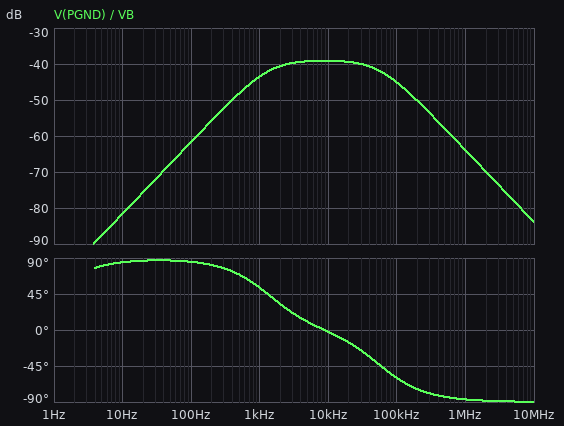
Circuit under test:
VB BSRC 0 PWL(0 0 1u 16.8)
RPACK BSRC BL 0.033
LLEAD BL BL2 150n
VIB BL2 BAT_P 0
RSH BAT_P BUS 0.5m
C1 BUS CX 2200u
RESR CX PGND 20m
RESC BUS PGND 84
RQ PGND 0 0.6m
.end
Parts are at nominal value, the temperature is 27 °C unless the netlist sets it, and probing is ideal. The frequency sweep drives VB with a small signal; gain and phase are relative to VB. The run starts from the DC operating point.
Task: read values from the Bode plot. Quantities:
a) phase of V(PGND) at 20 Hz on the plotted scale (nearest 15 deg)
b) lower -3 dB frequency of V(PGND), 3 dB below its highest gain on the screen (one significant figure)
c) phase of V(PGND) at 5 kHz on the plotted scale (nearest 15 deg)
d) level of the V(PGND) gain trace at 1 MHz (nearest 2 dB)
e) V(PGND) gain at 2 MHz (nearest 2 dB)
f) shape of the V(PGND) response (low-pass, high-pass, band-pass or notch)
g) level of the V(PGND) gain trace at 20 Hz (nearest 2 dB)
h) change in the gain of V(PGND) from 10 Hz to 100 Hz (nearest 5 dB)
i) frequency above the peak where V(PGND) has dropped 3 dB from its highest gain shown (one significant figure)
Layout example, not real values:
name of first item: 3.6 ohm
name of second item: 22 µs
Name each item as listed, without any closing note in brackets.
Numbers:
phase of V(PGND) at 20 Hz on the plotted scale: 90 deg
lower -3 dB frequency of V(PGND), 3 dB below its highest gain on the screen: 1 kHz
phase of V(PGND) at 5 kHz on the plotted scale: 15 deg
level of the V(PGND) gain trace at 1 MHz: -64 dB
V(PGND) gain at 2 MHz: -70 dB
shape of the V(PGND) response: band-pass
level of the V(PGND) gain trace at 20 Hz: -76 dB
change in the gain of V(PGND) from 10 Hz to 100 Hz: 20 dB
frequency above the peak where V(PGND) has dropped 3 dB from its highest gain shown: 60 kHz
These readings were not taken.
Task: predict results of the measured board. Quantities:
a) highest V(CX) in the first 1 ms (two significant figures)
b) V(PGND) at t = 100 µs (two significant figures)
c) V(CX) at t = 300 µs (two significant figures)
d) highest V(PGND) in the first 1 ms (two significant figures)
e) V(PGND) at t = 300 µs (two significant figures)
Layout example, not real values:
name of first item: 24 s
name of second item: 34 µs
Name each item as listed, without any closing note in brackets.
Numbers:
highest V(CX) in the first 1 ms: 6.0 V
V(PGND) at t = 100 µs: 83 mV
V(CX) at t = 300 µs: 510 mV
highest V(PGND) in the first 1 ms: 170 mV
V(PGND) at t = 300 µs: 15 mV
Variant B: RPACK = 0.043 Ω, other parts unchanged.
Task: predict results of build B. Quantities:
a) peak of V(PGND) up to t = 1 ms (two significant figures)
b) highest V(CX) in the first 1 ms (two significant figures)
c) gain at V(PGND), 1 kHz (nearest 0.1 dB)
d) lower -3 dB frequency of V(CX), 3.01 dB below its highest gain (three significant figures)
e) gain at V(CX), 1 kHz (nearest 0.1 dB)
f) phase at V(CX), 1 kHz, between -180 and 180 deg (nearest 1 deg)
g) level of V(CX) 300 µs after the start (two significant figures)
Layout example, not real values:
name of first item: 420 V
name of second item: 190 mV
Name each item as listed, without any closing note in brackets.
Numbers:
peak of V(PGND) up to t = 1 ms: 150 mV
highest V(CX) in the first 1 ms: 5.1 V
gain at V(PGND), 1 kHz: -44.1 dB
lower -3 dB frequency of V(CX), 3.01 dB below its highest gain: 1.11 kHz
gain at V(CX), 1 kHz: -13.4 dB
phase at V(CX), 1 kHz, between -180 and 180 deg: 48 deg
level of V(CX) 300 µs after the start: 640 mV
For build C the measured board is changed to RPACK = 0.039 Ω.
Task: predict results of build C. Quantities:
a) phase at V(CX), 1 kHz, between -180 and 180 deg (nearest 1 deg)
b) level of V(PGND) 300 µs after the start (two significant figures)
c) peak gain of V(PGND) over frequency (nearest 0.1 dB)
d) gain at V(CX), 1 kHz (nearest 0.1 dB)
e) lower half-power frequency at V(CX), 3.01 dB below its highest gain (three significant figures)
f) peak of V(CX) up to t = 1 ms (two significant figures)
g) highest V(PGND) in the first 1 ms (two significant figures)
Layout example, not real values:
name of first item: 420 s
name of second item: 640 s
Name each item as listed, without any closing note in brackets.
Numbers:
phase at V(CX), 1 kHz, between -180 and 180 deg: 50 deg
level of V(PGND) 300 µs after the start: 17 mV
peak gain of V(PGND) over frequency: -40.0 dB
gain at V(CX), 1 kHz: -13.1 dB
lower half-power frequency at V(CX), 3.01 dB below its highest gain: 1.18 kHz
peak of V(CX) up to t = 1 ms: 5.4 V
highest V(PGND) in the first 1 ms: 160 mV
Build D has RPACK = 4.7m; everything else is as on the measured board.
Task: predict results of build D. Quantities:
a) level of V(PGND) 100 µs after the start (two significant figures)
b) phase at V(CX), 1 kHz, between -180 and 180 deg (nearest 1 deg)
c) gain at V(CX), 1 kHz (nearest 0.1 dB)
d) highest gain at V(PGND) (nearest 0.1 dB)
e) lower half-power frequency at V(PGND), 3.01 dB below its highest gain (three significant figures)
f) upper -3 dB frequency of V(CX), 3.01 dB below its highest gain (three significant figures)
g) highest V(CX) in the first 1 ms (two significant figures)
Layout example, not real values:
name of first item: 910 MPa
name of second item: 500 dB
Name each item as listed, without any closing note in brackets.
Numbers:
level of V(PGND) 100 µs after the start: 70 mV
phase at V(CX), 1 kHz, between -180 and 180 deg: 70 deg
gain at V(CX), 1 kHz: -11.3 dB
highest gain at V(PGND): -32.7 dB
lower half-power frequency at V(PGND), 3.01 dB below its highest gain: 2.56 kHz
upper -3 dB frequency of V(CX), 3.01 dB below its highest gain: 29.9 kHz
highest V(CX) in the first 1 ms: 11 V
